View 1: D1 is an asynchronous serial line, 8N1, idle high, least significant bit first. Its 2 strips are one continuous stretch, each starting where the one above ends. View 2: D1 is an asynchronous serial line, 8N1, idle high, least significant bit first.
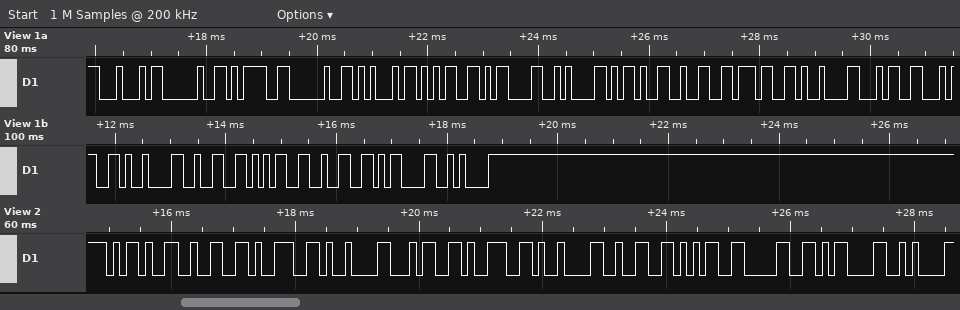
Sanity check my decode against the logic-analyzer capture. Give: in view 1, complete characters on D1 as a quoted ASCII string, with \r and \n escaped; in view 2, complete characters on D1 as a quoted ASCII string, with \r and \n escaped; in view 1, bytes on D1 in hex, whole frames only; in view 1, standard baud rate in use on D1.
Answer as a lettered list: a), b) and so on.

a) "D = E5\r\n-27\t44\t252\r\n"
b) "-29\t49\t250\r\n"
c) 44 20 3D 20 45 35 0D 0A 2D 32 37 09 34 34 09 32 35 32 0D 0A
d) 9600 baud
